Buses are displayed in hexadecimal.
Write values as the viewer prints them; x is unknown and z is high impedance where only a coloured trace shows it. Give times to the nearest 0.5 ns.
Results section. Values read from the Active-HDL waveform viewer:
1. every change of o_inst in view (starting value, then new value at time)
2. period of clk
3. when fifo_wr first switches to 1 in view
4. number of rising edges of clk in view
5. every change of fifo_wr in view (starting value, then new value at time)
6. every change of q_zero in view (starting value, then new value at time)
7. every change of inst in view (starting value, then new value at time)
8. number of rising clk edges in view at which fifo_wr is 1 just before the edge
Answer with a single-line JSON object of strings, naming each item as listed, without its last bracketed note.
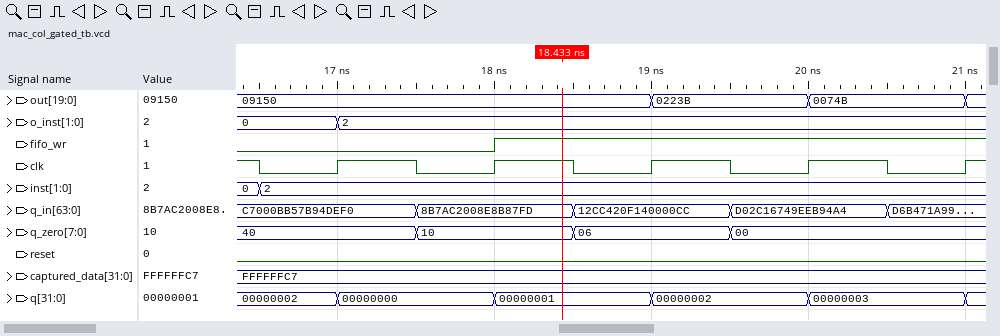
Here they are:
{"every change of o_inst in view": "0, 2 at 17 ns", "period of clk": "1 ns", "when fifo_wr first switches to 1 in view": "18 ns", "number of rising edges of clk in view": "5", "every change of fifo_wr in view": "0, 1 at 18 ns", "every change of q_zero in view": "40, 10 at 17.5 ns, 06 at 18.5 ns, 00 at 19.5 ns", "every change of inst in view": "0, 2 at 16.5 ns", "number of rising clk edges in view at which fifo_wr is 1 just before the edge": "3"}
